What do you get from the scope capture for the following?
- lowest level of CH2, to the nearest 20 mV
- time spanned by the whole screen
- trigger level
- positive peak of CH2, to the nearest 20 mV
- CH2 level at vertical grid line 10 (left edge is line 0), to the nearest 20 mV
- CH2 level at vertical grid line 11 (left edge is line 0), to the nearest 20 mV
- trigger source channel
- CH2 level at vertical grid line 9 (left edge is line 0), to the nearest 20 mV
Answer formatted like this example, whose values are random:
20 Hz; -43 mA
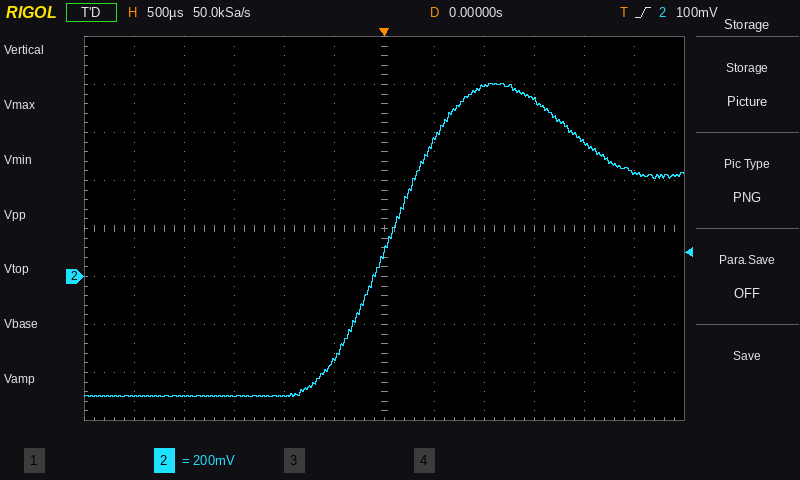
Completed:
-500 mV; 6 ms; 100 mV; 800 mV; 560 mV; 440 mV; CH2; 740 mV
